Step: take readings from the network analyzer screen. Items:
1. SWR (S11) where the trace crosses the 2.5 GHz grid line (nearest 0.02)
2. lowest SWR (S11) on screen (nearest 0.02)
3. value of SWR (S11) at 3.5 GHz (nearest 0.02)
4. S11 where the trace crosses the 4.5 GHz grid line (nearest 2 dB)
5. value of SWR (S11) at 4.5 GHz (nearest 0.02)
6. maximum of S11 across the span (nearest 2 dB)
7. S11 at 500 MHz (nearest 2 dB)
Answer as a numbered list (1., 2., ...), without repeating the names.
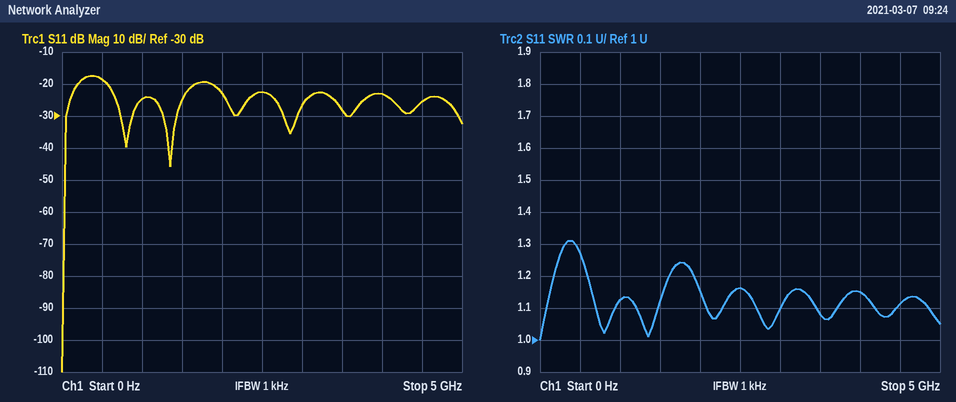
1. 1.16
2. 1.00
3. 1.08
4. -26 dB
5. 1.12
6. -18 dB
7. -18 dB
